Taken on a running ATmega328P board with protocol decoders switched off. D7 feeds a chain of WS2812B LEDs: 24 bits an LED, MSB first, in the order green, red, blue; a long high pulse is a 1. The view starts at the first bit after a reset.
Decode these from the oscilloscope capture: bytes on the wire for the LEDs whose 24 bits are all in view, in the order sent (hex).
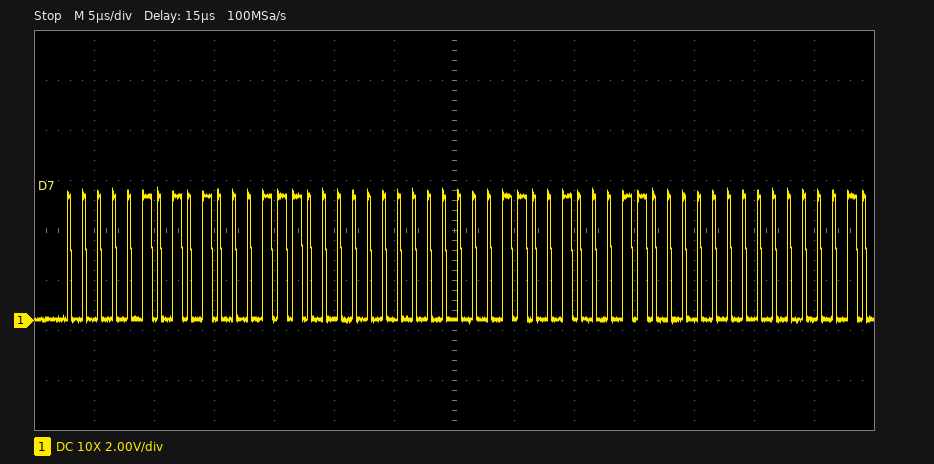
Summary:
05 47 00 06 46 00
